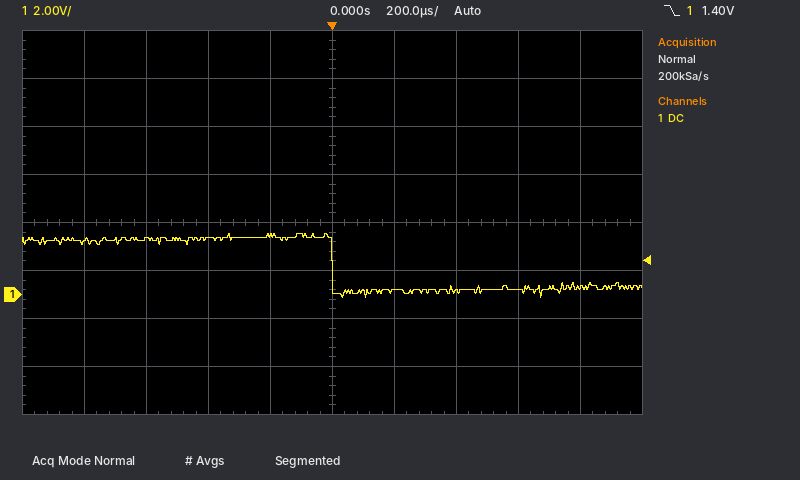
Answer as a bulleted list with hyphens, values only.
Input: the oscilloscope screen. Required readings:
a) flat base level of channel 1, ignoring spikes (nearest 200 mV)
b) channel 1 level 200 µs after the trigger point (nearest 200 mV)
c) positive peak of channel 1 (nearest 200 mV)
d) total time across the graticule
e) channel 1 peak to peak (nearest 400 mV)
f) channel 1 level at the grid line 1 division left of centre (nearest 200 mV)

- 200 mV
- 200 mV
- 2.6 V
- 2 ms
- 2.8 V
- 2.4 V
